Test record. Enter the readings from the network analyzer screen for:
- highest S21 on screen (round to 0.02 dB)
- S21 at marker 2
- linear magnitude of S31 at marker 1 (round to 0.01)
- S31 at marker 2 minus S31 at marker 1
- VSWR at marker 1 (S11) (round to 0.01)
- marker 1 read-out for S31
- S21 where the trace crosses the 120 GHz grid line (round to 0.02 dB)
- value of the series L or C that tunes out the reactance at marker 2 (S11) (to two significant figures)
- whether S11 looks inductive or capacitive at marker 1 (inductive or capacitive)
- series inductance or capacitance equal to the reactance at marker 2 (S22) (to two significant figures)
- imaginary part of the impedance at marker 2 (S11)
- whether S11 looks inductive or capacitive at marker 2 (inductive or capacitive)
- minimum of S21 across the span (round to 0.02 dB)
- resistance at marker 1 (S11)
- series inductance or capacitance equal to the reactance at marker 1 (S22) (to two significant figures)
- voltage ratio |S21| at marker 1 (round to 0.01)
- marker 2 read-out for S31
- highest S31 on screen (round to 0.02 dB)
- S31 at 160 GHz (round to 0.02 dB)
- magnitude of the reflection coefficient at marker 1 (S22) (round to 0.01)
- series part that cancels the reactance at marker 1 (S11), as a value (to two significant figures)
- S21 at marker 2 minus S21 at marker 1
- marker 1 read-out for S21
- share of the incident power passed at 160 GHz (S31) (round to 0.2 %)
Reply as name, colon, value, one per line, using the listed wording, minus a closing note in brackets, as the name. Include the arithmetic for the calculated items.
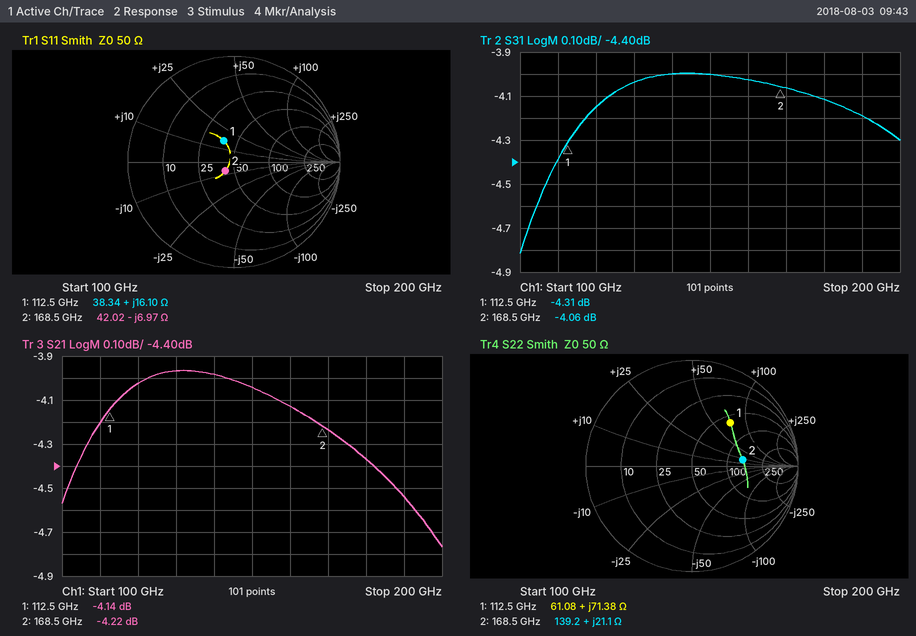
highest S21 on screen: -3.96 dB
S21 at marker 2: -4.22 dB
linear magnitude of S31 at marker 1: 10^(-4.31/20) ≈ 0.61
S31 at marker 2 minus S31 at marker 1: -4.06 − (-4.31) = 0.25 dB
VSWR at marker 1 (S11): 1.57
marker 1 read-out for S31: -4.31 dB
S21 where the trace crosses the 120 GHz grid line: -4.02 dB
value of the series L or C that tunes out the reactance at marker 2 (S11): L = 6.97 Ω/(2π × 168.5 GHz) ≈ 6.6 pH
whether S11 looks inductive or capacitive at marker 1: inductive
series inductance or capacitance equal to the reactance at marker 2 (S22): L = 21.1 Ω/(2π × 168.5 GHz) ≈ 20 pH
imaginary part of the impedance at marker 2: -6.97 Ω
whether S11 looks inductive or capacitive at marker 2: capacitive
minimum of S21 across the span: -4.76 dB
resistance at marker 1: 38.34 Ω
series inductance or capacitance equal to the reactance at marker 1 (S22): L = 71.38 Ω/(2π × 112.5 GHz) ≈ 101 pH, so 100 pH to two significant figures
voltage ratio |S21| at marker 1: 10^(-4.14/20) ≈ 0.62
marker 2 read-out for S31: -4.06 dB
highest S31 on screen: -4.00 dB
S31 at 160 GHz: -4.02 dB
magnitude of the reflection coefficient at marker 1 (S22): 0.55
series part that cancels the reactance at marker 1 (S11), as a value: C = 1/(2π × 112.5 GHz × 16.1 Ω) ≈ 88 fF
S21 at marker 2 minus S21 at marker 1: -4.22 − (-4.14) = -0.08 dB
marker 1 read-out for S21: -4.14 dB
share of the incident power passed at 160 GHz (S31): 10^(-4.02/10) ≈ 39.6 %
